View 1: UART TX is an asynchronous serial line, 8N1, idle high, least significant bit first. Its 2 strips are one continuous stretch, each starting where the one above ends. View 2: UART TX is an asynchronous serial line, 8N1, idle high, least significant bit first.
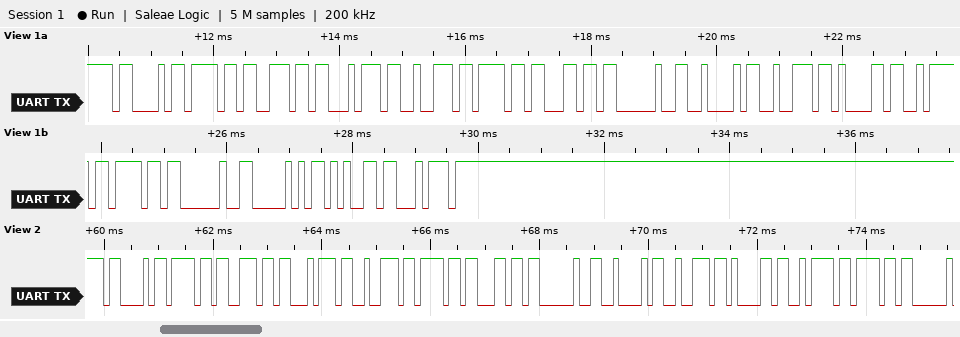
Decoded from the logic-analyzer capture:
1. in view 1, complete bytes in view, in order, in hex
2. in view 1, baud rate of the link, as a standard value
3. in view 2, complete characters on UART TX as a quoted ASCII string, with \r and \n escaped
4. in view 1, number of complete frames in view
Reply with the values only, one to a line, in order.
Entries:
43 6F 6E 74 72 6F 6C 20 42 72 61 7A 6F 20 50 65 74
9600 baud
"Control Brazo"
17
